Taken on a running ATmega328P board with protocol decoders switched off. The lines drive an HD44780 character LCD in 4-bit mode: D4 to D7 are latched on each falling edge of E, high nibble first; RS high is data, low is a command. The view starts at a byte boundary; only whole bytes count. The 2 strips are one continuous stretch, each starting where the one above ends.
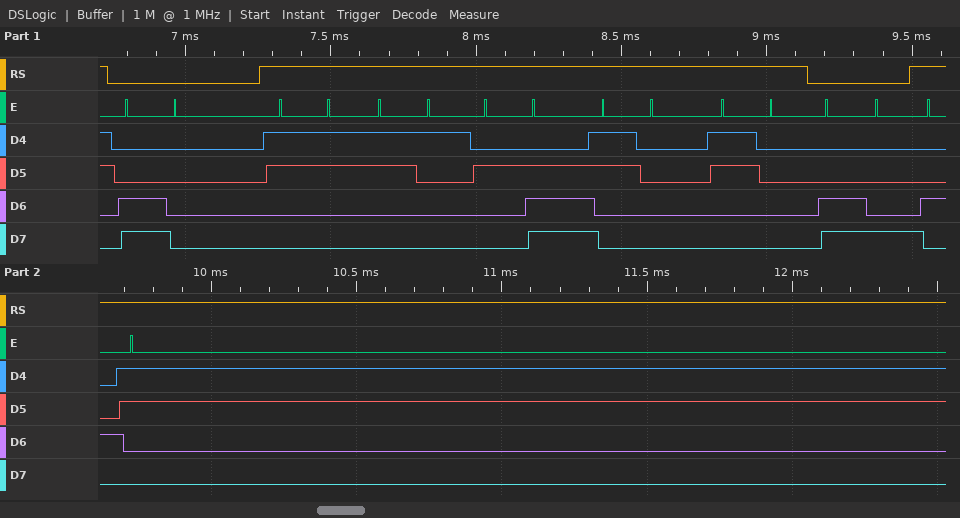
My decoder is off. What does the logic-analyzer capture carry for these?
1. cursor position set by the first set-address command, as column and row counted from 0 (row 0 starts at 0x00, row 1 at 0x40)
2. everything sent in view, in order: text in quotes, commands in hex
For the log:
column 0, row 1
0xC0 "31.00" 0xC8 "C"
